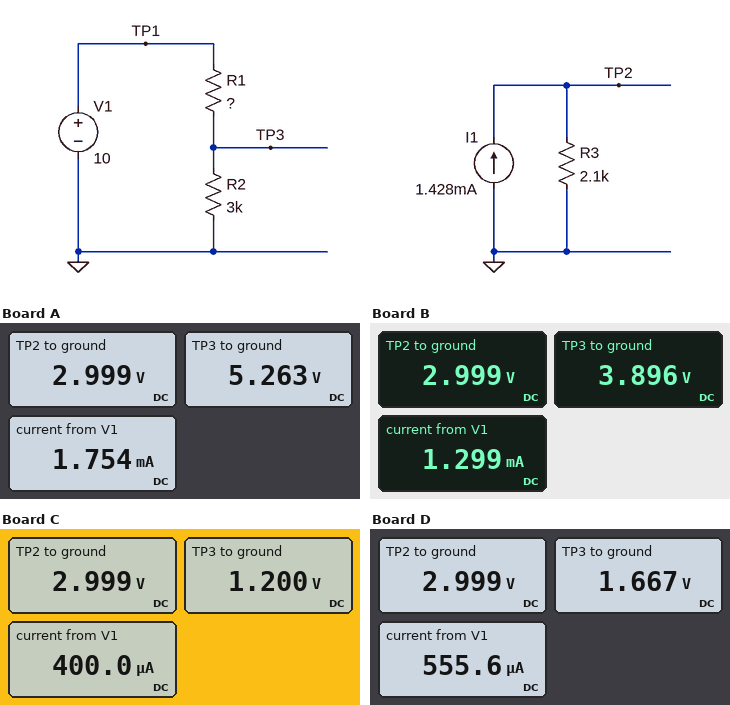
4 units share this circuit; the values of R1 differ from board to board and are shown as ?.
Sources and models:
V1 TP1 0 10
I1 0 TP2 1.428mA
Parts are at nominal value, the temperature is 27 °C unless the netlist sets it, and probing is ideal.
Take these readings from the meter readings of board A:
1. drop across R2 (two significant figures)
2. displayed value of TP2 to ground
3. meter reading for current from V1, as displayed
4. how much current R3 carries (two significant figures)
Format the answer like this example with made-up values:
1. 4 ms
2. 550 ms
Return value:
1. 5.3 V
2. 2.999 V
3. 1.754 mA
4. 1.4 mA
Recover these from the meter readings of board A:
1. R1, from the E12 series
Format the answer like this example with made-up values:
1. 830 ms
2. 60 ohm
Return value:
1. 2.7 kΩ
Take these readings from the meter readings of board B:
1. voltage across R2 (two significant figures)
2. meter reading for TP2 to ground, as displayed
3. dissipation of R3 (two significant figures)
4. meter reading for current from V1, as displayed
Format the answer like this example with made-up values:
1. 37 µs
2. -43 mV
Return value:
1. 3.9 V
2. 2.999 V
3. 4.3 mW
4. 1.299 mA
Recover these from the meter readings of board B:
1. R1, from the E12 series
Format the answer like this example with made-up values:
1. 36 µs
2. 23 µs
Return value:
1. 4.7 kΩ
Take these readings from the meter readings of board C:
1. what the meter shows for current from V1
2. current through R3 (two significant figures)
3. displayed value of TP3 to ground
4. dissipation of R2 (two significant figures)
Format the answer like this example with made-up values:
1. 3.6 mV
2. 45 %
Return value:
1. 400.0 µA
2. 1.4 mA
3. 1.200 V
4. 480 µW
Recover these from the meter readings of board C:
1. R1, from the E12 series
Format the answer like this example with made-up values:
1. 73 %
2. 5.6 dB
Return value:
1. 22 kΩ
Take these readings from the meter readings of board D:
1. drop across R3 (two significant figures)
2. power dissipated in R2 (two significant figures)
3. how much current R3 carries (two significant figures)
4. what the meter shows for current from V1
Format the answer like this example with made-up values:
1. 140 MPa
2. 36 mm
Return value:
1. 3.0 V
2. 930 µW
3. 1.4 mA
4. 555.6 µA
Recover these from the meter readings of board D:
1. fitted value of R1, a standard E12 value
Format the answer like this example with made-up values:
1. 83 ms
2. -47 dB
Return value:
1. 15 kΩ
